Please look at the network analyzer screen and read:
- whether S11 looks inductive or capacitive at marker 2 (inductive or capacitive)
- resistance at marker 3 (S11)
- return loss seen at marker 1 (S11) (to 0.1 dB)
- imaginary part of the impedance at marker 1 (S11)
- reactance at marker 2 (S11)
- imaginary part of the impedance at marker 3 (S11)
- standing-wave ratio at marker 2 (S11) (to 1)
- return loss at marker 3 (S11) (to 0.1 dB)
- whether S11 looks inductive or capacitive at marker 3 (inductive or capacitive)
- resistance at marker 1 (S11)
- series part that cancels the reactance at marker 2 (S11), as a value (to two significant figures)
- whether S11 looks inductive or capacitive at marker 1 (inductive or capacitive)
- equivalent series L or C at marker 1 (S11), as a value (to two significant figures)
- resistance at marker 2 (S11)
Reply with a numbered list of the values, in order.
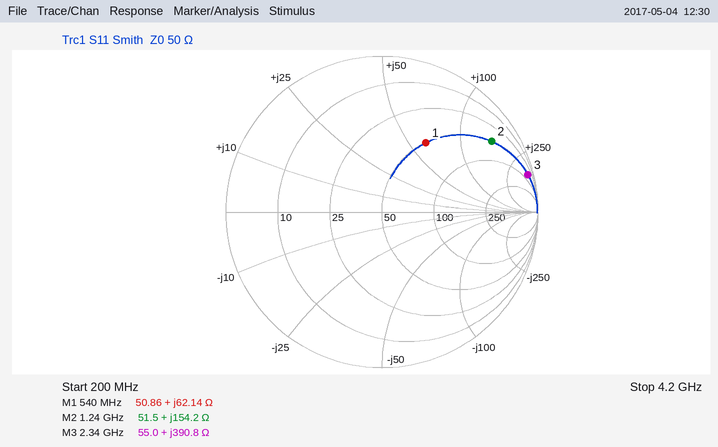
1. inductive
2. 55.0 Ω
3. 5.6 dB
4. +62.14 Ω
5. +154.2 Ω
6. +390.8 Ω
7. 11
8. 0.3 dB
9. inductive
10. 50.86 Ω
11. 830 fF
12. inductive
13. 18 nH
14. 51.5 Ω
